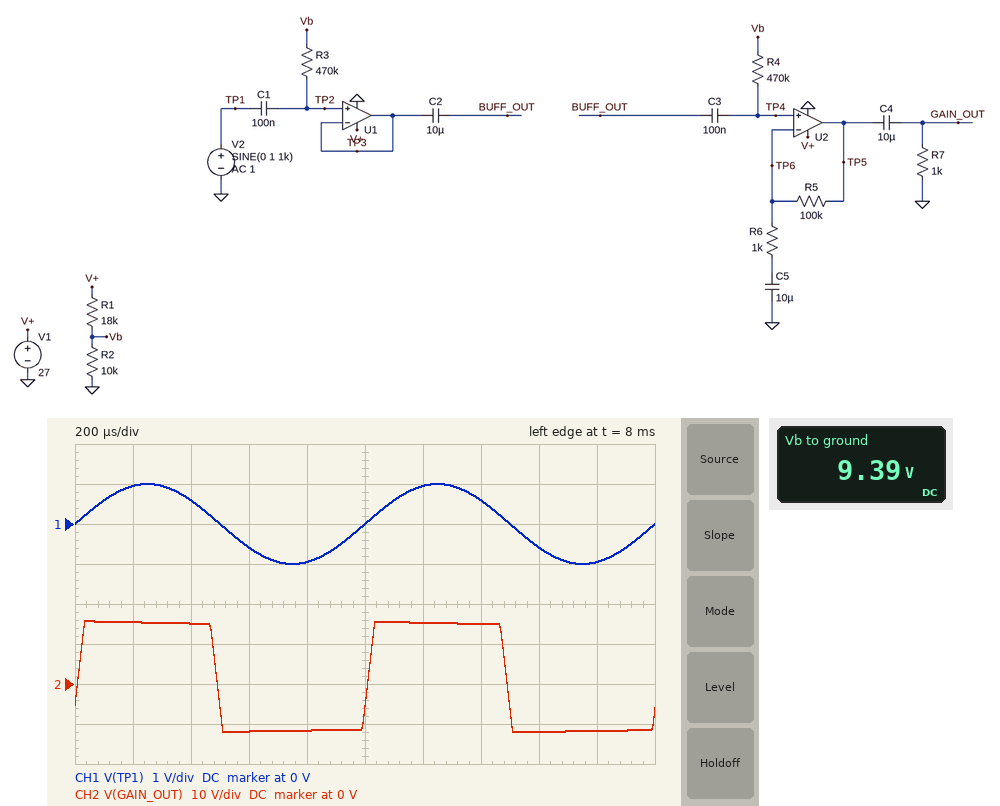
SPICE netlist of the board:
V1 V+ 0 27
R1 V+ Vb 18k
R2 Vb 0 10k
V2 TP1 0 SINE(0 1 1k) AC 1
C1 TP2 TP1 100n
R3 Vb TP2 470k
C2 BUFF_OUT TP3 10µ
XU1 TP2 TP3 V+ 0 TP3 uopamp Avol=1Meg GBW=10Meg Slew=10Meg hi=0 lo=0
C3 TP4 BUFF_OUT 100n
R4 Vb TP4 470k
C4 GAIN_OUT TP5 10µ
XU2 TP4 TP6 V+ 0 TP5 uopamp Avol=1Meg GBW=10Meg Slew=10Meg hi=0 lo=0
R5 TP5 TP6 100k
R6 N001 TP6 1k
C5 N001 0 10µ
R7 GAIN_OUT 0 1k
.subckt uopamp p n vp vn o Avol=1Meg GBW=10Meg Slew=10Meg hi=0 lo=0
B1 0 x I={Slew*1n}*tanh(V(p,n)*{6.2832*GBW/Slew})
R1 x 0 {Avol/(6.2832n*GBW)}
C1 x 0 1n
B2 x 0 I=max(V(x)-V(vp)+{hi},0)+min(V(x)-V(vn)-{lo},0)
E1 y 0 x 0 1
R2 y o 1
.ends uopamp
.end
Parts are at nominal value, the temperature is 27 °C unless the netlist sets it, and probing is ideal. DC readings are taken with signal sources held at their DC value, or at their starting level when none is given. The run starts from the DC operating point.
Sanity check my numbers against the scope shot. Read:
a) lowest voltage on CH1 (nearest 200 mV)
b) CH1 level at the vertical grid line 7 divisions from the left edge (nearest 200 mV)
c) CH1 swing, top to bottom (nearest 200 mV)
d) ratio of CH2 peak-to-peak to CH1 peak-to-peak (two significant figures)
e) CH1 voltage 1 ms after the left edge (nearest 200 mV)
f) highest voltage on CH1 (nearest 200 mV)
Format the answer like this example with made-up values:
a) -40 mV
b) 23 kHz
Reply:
a) -1.0 V
b) 600 mV
c) 2.0 V
d) 14
e) 0 V
f) 1.0 V
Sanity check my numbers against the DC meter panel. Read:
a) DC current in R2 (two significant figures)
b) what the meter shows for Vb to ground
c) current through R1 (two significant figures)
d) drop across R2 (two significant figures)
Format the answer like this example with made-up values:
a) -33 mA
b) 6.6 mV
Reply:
a) 940 µA
b) 9.39 V
c) 980 µA
d) 9.4 V
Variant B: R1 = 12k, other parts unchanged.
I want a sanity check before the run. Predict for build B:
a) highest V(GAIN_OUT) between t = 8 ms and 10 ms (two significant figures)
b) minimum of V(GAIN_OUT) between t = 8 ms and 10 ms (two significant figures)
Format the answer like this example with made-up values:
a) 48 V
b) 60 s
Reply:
a) 14 V
b) -13 V
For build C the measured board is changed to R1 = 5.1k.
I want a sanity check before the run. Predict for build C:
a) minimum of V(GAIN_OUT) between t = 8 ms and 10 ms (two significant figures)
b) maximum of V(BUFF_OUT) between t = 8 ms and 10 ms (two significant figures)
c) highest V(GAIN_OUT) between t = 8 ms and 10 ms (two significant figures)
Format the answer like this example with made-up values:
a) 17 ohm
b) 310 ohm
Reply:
a) -16 V
b) 1.0 V
c) 12 V
